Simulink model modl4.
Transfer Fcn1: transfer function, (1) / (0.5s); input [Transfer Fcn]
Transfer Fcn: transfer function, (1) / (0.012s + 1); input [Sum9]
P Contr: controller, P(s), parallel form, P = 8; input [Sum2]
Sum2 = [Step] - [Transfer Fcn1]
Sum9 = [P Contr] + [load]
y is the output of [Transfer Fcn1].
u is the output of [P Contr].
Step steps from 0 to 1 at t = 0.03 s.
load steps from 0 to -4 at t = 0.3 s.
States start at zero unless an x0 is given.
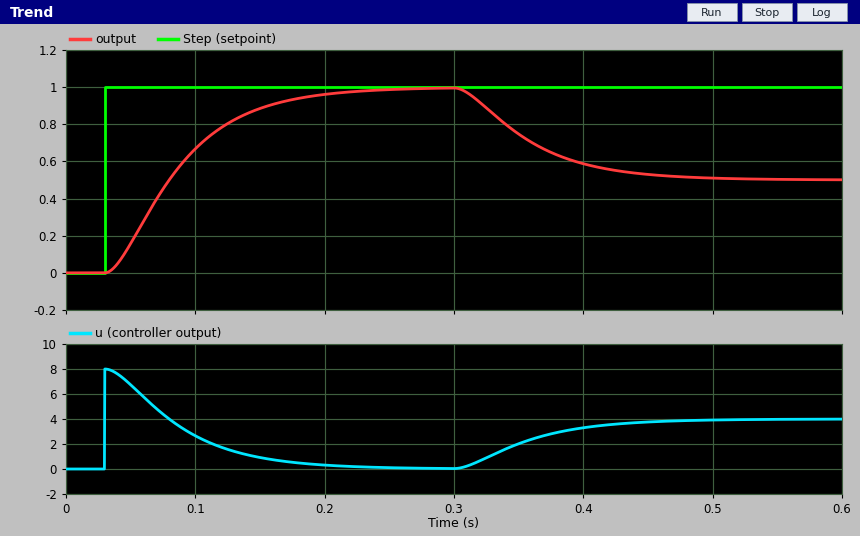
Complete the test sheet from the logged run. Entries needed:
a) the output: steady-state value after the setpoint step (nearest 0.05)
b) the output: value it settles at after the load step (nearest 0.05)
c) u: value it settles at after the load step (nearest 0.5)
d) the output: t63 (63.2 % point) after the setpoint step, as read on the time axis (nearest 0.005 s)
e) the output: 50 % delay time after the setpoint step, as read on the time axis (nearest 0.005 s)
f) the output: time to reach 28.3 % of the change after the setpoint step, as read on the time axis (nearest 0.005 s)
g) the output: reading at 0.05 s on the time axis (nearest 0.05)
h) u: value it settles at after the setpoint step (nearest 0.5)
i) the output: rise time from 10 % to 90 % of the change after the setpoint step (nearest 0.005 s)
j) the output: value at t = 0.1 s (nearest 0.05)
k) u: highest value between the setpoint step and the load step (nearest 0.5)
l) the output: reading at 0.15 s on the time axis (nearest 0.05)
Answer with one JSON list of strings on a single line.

["1.00", "0.50", "4.0", "0.095 s", "0.080 s", "0.060 s", "0.15", "0.0", "0.110 s", "0.65", "8.0", "0.90"]
